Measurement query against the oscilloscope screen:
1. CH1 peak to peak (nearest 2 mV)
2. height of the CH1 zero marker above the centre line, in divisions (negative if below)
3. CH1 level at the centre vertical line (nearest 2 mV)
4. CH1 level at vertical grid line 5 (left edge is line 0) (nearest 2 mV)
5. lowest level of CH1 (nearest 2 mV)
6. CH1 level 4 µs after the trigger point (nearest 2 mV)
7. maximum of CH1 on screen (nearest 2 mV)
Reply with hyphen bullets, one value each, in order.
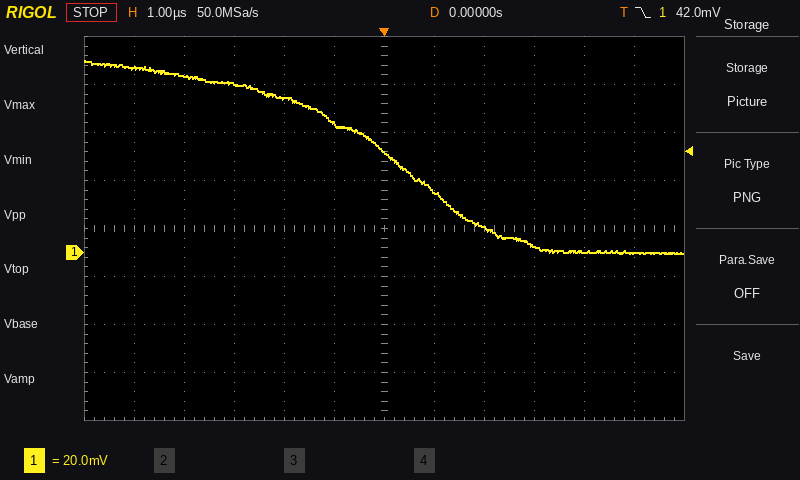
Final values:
- 80 mV
- -0.5 div
- 42 mV
- 54 mV
- 0 mV
- 0 mV
- 80 mV
